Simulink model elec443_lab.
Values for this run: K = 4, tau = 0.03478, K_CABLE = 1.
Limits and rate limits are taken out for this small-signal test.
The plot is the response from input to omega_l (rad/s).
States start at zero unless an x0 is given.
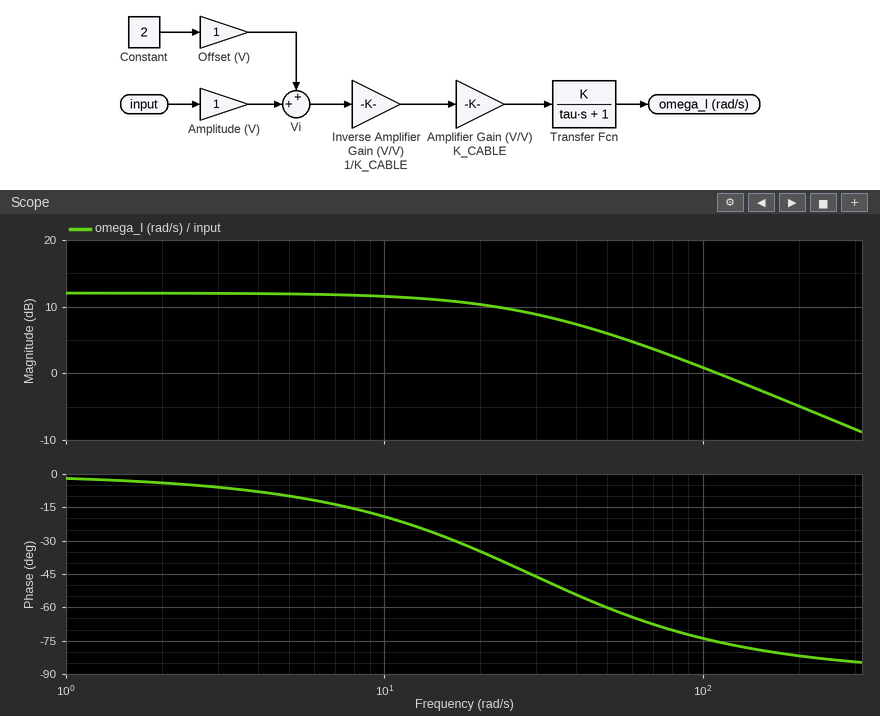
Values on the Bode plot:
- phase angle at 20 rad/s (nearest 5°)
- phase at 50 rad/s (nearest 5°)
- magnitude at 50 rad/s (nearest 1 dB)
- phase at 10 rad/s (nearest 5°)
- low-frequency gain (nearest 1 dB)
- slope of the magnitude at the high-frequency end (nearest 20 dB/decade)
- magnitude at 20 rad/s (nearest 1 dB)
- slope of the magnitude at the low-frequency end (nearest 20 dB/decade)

-35°
-60°
6 dB
-20°
12 dB
-20 dB/decade
10 dB
0 dB/decade
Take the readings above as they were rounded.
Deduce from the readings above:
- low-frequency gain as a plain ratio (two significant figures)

4.0
